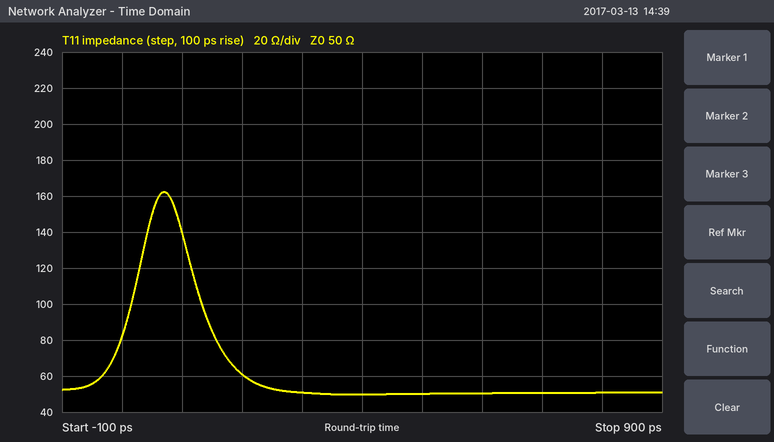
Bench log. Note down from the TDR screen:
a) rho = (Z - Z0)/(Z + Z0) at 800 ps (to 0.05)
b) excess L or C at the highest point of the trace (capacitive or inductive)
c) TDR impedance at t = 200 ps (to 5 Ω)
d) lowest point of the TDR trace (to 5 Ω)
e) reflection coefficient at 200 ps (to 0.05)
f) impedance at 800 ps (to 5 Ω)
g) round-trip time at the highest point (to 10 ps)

0.00
inductive
60 Ω
50 Ω
+0.10
50 Ω
70 ps
